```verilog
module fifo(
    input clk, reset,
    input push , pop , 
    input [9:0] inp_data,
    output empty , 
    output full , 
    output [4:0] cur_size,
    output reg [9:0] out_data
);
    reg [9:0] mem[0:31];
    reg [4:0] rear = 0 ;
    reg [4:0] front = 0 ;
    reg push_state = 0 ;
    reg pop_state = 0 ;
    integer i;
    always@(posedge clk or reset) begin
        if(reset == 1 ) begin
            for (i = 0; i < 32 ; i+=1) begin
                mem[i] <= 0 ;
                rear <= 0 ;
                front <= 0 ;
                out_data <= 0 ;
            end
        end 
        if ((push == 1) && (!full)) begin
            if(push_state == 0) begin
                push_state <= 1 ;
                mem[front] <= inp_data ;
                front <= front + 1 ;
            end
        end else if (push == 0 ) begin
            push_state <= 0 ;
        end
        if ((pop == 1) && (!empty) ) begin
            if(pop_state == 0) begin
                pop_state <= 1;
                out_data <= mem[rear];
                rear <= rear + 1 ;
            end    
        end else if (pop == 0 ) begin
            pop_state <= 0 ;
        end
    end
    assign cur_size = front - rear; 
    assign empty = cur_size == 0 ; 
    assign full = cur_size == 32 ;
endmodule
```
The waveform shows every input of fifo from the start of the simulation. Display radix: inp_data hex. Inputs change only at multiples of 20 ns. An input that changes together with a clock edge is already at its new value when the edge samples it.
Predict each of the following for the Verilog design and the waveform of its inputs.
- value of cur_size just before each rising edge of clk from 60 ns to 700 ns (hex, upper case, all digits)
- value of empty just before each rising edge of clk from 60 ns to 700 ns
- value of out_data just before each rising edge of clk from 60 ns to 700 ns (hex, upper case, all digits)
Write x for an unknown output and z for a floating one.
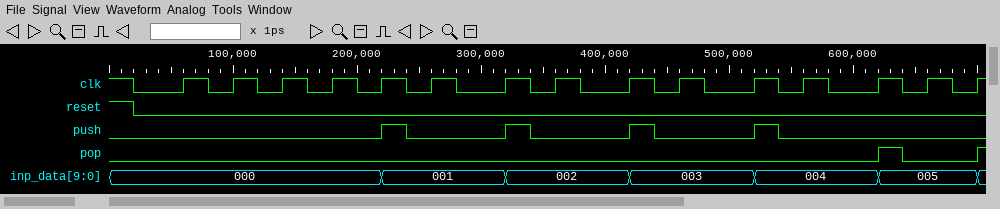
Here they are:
00, 00, 00, 00, 00, 01, 01, 02, 02, 03, 03, 04, 04, 03, 03
1 1 1 1 1 0 0 0 0 0 0 0 0 0 0
000, 000, 000, 000, 000, 000, 000, 000, 000, 000, 000, 000, 000, 001, 001
